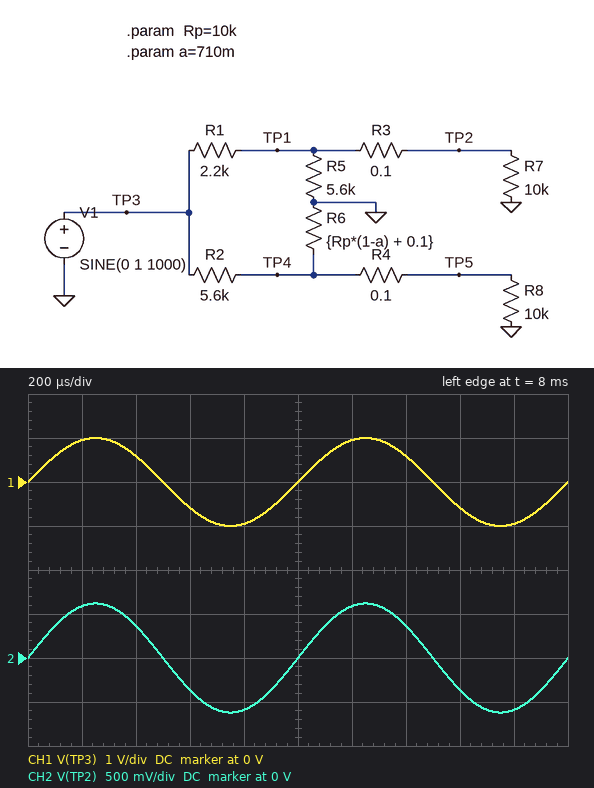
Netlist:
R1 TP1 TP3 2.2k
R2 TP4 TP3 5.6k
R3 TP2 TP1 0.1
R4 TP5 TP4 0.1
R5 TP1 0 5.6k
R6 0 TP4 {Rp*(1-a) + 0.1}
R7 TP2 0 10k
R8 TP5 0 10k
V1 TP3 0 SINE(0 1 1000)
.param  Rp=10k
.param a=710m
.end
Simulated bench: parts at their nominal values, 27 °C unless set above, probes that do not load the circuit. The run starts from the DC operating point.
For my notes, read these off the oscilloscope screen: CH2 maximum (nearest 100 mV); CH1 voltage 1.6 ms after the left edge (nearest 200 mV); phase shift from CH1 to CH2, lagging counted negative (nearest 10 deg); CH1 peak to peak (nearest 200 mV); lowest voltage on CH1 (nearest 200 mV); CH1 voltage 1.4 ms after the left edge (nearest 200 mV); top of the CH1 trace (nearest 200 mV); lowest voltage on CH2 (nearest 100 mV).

600 mV
-600 mV
0 deg
2.0 V
-1.0 V
600 mV
1.0 V
-600 mV
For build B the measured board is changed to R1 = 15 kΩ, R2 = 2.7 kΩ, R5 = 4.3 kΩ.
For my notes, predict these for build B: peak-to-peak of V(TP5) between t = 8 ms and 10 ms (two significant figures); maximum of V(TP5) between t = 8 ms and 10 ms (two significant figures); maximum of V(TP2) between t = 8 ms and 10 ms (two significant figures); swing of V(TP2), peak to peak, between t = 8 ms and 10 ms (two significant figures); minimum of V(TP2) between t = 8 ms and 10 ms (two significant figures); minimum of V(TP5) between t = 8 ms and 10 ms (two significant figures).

910 mV
450 mV
170 mV
330 mV
-170 mV
-450 mV
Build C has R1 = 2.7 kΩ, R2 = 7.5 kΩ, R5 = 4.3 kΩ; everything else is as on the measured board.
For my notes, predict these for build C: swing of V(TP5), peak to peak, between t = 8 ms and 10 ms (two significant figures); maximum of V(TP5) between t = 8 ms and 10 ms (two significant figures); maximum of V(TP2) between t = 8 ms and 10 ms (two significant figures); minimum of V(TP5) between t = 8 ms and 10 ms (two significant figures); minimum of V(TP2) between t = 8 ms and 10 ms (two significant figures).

460 mV
230 mV
530 mV
-230 mV
-530 mV
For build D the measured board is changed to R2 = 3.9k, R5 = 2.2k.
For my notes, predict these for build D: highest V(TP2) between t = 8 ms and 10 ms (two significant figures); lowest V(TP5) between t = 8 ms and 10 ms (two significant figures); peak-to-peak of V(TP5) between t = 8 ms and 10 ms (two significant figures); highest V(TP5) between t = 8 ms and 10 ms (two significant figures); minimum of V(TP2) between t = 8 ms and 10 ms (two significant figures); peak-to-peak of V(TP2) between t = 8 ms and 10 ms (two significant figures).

450 mV
-370 mV
730 mV
370 mV
-450 mV
900 mV
